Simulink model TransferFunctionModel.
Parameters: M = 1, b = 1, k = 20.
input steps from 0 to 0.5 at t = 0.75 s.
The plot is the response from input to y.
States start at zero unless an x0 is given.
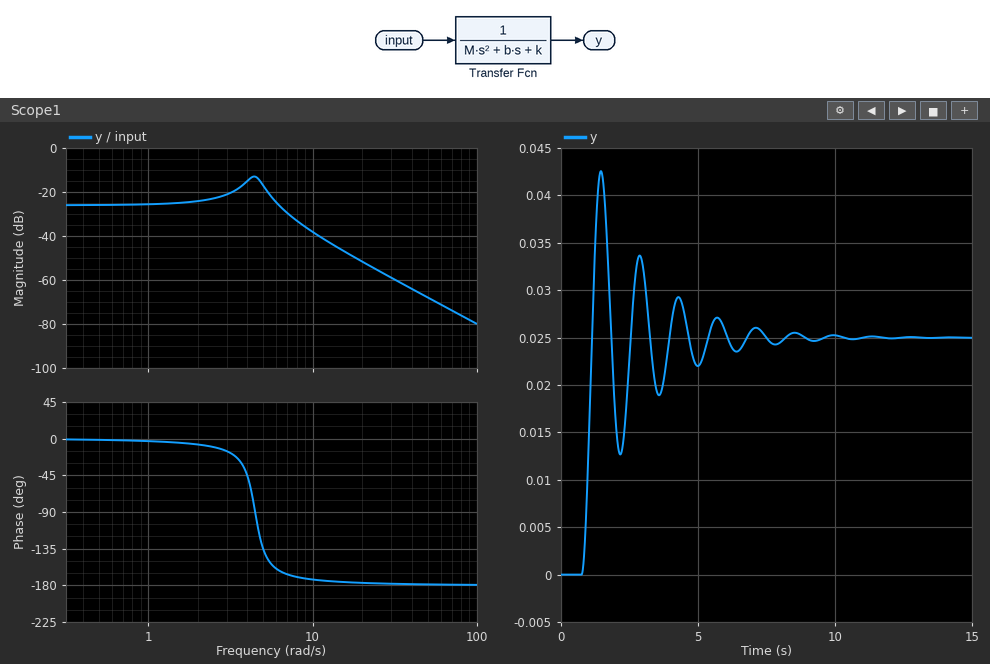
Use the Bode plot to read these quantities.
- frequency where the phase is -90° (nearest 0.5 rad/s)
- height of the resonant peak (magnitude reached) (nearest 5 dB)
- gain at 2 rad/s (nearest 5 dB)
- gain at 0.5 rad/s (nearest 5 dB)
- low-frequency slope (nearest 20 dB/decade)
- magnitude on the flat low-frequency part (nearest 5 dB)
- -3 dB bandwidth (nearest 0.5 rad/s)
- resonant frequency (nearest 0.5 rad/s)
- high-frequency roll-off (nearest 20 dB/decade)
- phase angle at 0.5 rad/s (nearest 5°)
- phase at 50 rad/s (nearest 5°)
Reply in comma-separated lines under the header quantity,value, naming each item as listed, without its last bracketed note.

quantity,value
frequency where the phase is -90°,4.5 rad/s
height of the resonant peak (magnitude reached),-15 dB
gain at 2 rad/s,-25 dB
gain at 0.5 rad/s,-25 dB
low-frequency slope,0 dB/decade
magnitude on the flat low-frequency part,-25 dB
-3 dB bandwidth,7.0 rad/s
resonant frequency,4.5 rad/s
high-frequency roll-off,-40 dB/decade
phase angle at 0.5 rad/s,0°
phase at 50 rad/s,-180°
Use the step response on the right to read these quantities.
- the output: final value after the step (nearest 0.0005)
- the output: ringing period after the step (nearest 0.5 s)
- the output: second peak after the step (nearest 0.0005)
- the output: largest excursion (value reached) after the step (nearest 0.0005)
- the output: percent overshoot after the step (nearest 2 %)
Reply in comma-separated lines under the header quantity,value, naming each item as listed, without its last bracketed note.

quantity,value
the output: final value after the step,0.0250
the output: ringing period after the step,1.5 s
the output: second peak after the step,0.0335
the output: largest excursion (value reached) after the step,0.0425
the output: percent overshoot after the step,70 %
